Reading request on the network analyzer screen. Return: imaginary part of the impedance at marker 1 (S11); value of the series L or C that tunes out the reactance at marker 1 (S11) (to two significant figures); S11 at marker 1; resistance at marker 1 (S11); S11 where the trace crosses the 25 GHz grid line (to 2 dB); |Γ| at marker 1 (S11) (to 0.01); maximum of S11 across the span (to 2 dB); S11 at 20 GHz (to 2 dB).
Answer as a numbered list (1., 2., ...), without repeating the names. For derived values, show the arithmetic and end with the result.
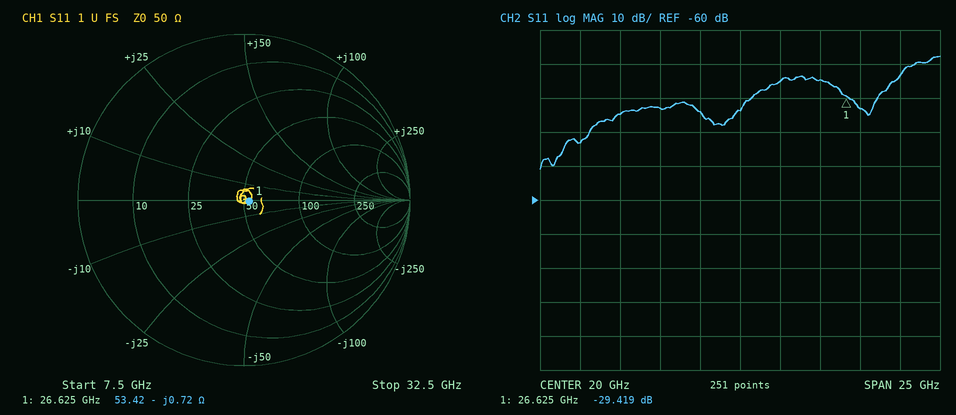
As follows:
1. -0.72 Ω
2. L = 0.72 Ω/(2π × 26.625 GHz) ≈ 4.3 pH
3. -29.419 dB
4. 53.42 Ω
5. -24 dB
6. 0.03
7. -18 dB
8. -34 dB
